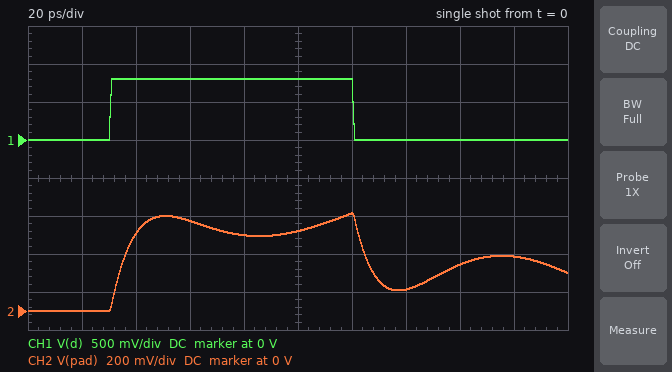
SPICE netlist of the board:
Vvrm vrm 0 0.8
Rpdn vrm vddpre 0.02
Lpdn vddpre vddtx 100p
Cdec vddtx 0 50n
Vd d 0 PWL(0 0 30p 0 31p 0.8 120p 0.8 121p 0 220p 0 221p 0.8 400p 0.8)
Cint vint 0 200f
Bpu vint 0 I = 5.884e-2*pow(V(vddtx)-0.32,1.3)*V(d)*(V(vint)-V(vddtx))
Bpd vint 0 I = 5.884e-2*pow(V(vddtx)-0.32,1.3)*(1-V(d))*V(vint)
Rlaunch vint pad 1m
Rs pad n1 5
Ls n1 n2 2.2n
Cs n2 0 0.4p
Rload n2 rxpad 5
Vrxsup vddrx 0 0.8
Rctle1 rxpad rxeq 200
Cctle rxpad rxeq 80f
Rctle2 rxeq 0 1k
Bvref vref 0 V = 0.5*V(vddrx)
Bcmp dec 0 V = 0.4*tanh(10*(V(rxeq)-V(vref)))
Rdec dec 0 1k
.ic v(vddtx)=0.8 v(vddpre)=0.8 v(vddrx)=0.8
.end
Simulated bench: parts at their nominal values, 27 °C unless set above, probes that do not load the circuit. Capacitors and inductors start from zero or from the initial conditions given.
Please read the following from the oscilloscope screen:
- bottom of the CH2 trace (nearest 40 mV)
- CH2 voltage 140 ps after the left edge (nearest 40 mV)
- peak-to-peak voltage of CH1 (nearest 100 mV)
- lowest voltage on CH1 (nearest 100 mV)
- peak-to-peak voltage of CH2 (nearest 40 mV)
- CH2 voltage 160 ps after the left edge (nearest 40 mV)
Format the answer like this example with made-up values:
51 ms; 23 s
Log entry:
0 V; 120 mV; 800 mV; 0 V; 520 mV; 240 mV
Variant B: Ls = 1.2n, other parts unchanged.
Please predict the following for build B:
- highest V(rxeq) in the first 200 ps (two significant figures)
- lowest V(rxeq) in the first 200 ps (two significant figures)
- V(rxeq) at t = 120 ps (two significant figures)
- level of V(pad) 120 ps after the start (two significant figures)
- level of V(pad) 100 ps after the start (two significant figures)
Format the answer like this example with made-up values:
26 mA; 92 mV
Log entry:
600 mV; -95 mV; 570 mV; 630 mV; 500 mV
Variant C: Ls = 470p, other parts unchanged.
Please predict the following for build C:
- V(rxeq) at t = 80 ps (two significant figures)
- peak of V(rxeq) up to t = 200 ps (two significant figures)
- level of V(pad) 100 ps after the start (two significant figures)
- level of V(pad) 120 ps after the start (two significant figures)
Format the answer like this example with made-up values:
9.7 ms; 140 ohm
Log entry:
490 mV; 510 mV; 610 mV; 590 mV
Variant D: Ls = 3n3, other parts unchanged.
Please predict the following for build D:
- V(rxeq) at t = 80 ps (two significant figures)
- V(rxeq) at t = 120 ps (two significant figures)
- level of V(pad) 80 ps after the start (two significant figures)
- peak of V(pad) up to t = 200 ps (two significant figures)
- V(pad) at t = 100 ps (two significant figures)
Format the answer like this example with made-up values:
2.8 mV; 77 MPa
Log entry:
280 mV; 620 mV; 450 mV; 530 mV; 420 mV
